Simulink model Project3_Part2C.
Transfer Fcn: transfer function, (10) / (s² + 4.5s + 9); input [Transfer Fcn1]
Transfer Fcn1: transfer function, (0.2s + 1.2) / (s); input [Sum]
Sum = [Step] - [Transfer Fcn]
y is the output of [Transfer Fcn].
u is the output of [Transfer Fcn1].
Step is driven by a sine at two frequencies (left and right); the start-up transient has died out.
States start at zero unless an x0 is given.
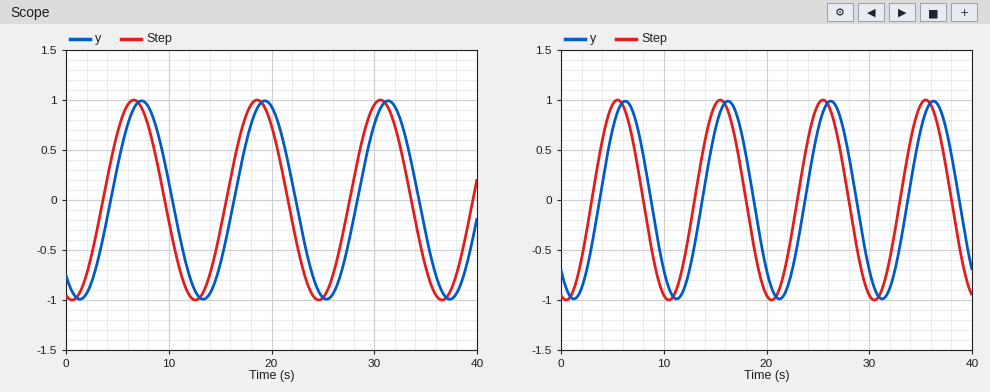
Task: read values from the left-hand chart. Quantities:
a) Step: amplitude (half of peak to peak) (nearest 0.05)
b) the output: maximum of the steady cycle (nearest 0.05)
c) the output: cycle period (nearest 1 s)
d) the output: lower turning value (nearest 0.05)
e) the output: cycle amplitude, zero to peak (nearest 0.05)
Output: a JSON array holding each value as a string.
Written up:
["1.00", "1.00", "12 s", "-1.00", "1.00"]
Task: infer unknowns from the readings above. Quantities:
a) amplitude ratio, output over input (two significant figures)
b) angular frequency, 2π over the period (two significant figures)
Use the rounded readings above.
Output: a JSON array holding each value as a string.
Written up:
["1.0", "0.52 rad/s"]
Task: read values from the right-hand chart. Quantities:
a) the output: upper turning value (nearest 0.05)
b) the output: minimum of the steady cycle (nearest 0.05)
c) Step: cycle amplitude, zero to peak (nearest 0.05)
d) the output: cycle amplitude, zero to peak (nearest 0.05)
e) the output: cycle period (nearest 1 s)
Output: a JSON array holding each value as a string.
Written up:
["1.00", "-1.00", "1.00", "1.00", "10 s"]
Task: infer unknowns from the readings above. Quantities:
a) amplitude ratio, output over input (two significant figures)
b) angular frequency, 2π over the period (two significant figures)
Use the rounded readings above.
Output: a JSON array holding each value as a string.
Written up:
["1.0", "0.63 rad/s"]
